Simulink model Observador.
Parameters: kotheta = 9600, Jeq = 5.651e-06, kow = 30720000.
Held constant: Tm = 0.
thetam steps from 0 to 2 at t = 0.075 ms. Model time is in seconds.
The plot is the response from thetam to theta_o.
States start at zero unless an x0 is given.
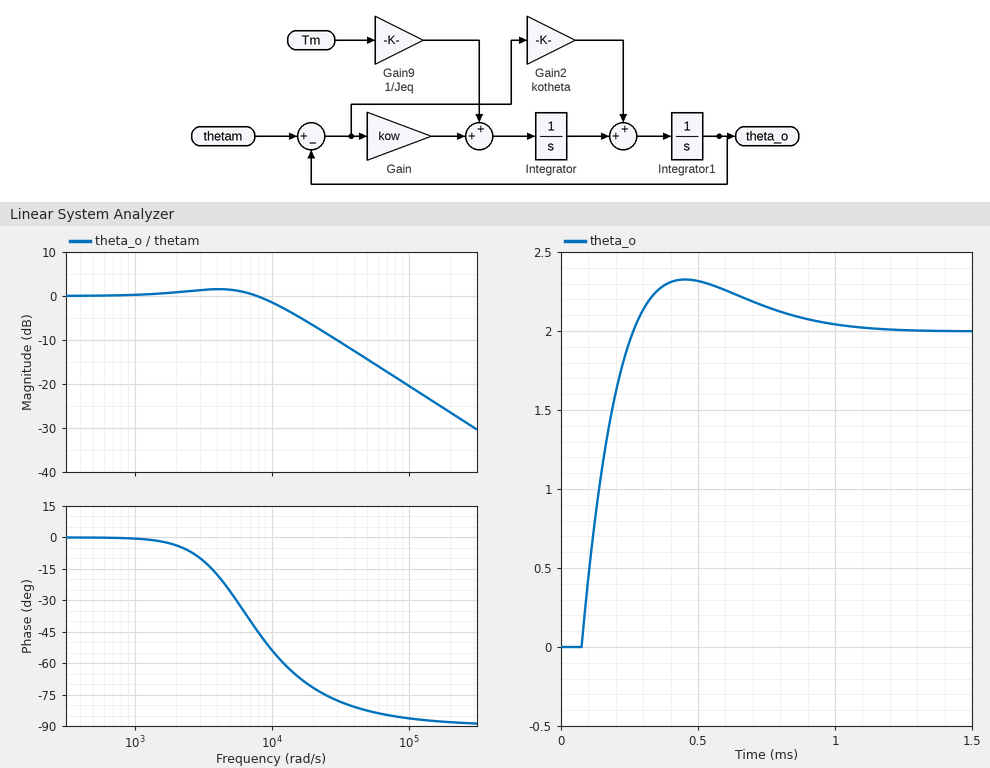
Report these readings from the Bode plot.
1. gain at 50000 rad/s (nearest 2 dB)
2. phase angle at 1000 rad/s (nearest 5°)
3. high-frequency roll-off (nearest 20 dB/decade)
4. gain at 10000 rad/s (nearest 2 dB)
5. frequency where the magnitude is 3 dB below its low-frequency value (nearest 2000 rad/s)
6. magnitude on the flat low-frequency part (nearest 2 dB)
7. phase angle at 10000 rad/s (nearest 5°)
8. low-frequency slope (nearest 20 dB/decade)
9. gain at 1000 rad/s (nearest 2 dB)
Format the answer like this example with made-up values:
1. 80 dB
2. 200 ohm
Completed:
1. -14 dB
2. 0°
3. -20 dB/decade
4. -2 dB
5. 12000 rad/s
6. 0 dB
7. -55°
8. 0 dB/decade
9. 0 dB
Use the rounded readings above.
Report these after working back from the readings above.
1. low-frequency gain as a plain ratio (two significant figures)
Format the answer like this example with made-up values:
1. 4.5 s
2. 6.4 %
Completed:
1. 1.0
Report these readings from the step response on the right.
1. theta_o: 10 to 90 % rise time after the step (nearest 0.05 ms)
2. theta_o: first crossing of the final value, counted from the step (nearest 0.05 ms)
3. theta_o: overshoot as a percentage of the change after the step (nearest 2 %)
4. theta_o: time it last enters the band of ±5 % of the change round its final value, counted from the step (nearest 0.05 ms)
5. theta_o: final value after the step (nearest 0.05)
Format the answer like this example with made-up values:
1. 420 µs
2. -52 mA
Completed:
1. 0.15 ms
2. 0.20 ms
3. 16 %
4. 0.75 ms
5. 2.00
